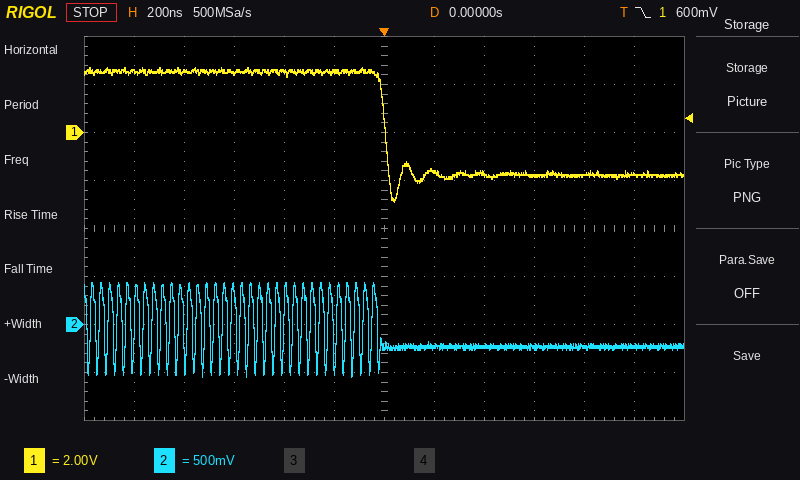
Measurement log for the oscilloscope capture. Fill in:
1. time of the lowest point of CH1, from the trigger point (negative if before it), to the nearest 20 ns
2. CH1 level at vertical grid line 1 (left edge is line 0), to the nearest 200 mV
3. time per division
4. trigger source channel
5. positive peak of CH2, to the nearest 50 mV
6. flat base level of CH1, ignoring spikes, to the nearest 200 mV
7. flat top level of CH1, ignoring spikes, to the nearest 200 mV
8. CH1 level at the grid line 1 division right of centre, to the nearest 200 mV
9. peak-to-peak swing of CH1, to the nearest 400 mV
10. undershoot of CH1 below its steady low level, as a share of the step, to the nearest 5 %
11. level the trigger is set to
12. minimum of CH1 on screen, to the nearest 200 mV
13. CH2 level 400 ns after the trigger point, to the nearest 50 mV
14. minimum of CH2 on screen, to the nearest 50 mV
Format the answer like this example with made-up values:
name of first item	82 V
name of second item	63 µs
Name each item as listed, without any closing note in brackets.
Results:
time of the lowest point of CH1, from the trigger point (negative if before it), to the nearest 20 ns	+40 ns
CH1 level at vertical grid line 1 (left edge is line 0), to the nearest 200 mV	2.6 V
time per division	200 ns
trigger source channel	CH1
positive peak of CH2, to the nearest 50 mV	450 mV
flat base level of CH1, ignoring spikes, to the nearest 200 mV	-1.8 V
flat top level of CH1, ignoring spikes, to the nearest 200 mV	2.6 V
CH1 level at the grid line 1 division right of centre, to the nearest 200 mV	-1.6 V
peak-to-peak swing of CH1, to the nearest 400 mV	5.6 V
undershoot of CH1 below its steady low level, as a share of the step, to the nearest 5 %	25 %
level the trigger is set to	600 mV
minimum of CH1 on screen, to the nearest 200 mV	-2.8 V
CH2 level 400 ns after the trigger point, to the nearest 50 mV	-200 mV
minimum of CH2 on screen, to the nearest 50 mV	-550 mV
